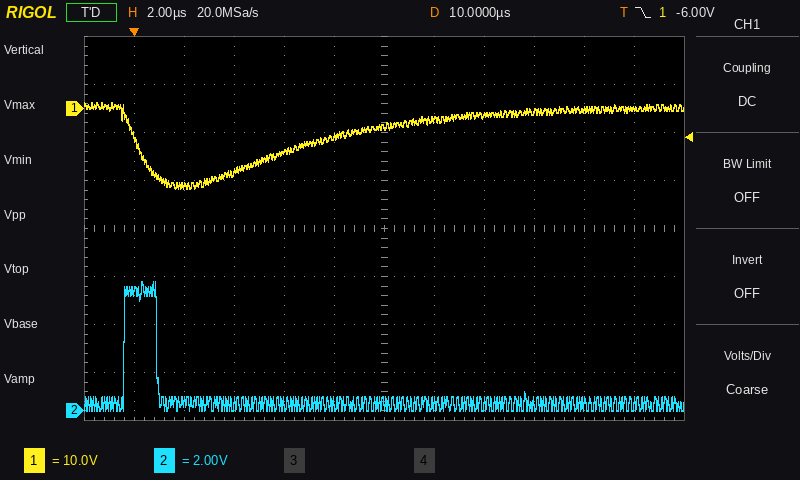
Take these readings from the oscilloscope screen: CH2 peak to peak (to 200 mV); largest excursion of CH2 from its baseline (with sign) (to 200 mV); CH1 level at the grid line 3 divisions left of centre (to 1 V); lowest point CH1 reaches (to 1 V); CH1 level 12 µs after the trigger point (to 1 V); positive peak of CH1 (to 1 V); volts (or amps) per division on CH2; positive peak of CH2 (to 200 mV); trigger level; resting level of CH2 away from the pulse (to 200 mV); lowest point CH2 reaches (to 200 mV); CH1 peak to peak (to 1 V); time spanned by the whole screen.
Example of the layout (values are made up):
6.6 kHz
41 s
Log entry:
5.4 V
+5.0 V
-13 V
-17 V
-2 V
1 V
2 V
5.4 V
-6.00 V
400 mV
0.0 V
18 V
24 µs
